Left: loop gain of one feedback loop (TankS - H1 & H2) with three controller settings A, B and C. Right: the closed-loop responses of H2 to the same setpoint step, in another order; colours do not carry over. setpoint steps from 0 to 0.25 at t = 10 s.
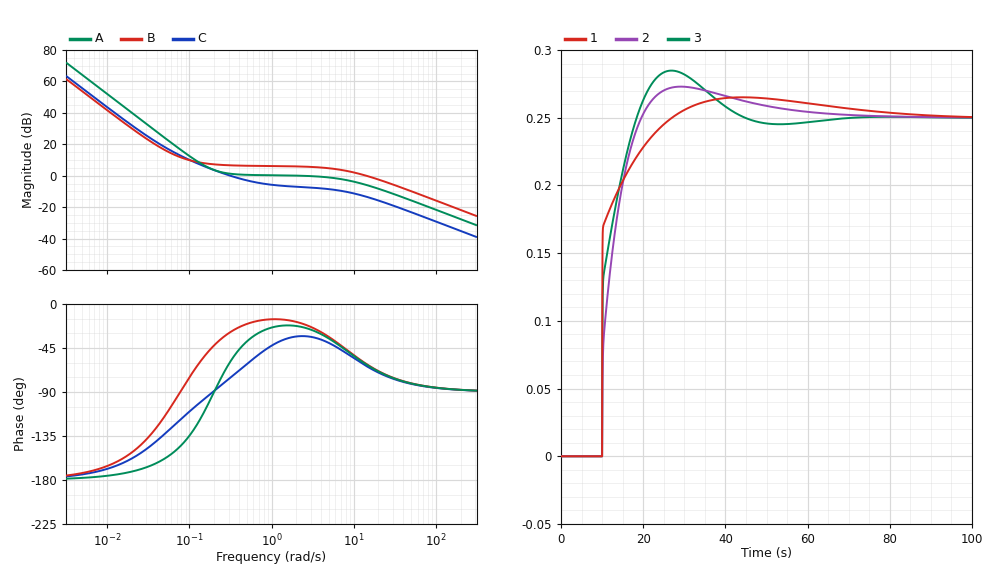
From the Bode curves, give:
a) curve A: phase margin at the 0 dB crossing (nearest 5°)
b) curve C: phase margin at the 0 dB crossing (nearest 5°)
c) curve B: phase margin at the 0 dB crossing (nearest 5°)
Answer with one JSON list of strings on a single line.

["155°", "105°", "120°"]
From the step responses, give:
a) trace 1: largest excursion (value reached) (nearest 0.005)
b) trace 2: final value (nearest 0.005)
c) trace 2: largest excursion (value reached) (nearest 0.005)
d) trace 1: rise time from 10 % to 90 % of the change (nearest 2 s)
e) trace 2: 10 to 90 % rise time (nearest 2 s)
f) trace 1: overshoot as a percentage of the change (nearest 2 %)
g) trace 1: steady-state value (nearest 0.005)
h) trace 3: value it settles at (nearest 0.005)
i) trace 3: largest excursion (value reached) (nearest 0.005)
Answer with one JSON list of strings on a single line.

["0.265", "0.250", "0.275", "10 s", "6 s", "6 %", "0.250", "0.250", "0.285"]
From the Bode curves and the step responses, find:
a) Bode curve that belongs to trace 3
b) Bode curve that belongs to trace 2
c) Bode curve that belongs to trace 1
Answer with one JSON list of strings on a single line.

["A", "C", "B"]
